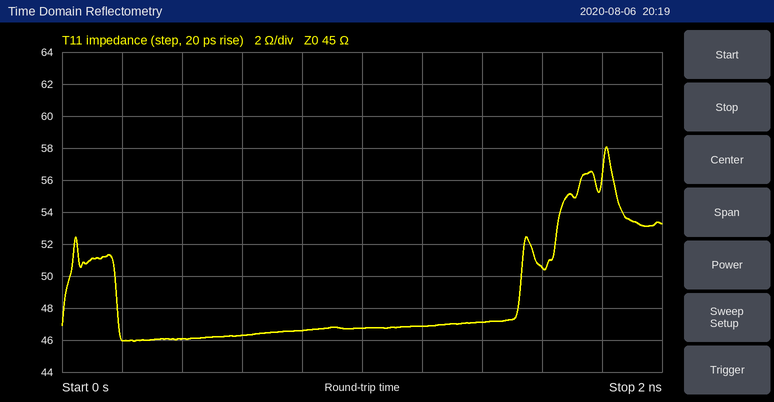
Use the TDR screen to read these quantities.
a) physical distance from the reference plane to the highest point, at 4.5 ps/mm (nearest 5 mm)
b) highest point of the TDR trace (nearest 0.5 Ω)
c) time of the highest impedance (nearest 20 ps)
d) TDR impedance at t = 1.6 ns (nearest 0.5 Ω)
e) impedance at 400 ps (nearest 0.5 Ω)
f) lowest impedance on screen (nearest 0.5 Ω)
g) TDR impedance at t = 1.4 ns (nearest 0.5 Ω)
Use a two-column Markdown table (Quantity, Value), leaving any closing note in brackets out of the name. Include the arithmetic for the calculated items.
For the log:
| Quantity | Value |
|---|---|
| physical distance from the reference plane to the highest point, at 4.5 ps/mm | 1.82 ns / 2 / 4.5 ps/mm ≈ 202 mm, so 200 mm to the nearest 5 mm |
| highest point of the TDR trace | 58.0 Ω |
| time of the highest impedance | 1.82 ns |
| TDR impedance at t = 1.6 ns | 50.5 Ω |
| impedance at 400 ps | 46.0 Ω |
| lowest impedance on screen | 46.0 Ω |
| TDR impedance at t = 1.4 ns | 47.0 Ω |
